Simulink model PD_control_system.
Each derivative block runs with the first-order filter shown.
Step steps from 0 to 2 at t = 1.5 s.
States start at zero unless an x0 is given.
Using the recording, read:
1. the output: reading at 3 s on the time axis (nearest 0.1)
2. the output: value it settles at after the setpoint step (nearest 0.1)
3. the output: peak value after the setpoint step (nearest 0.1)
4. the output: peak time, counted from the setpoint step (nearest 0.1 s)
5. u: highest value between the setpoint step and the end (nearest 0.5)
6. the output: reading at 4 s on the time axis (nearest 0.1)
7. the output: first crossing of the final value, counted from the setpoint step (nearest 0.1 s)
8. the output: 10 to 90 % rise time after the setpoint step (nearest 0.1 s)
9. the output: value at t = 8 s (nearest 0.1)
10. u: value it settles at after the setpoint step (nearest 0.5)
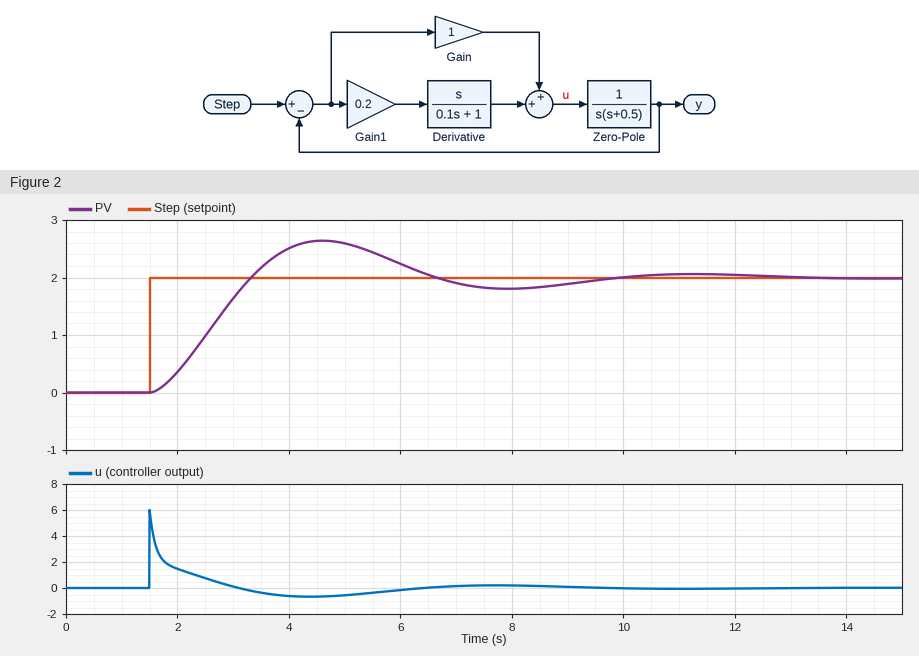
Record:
1.6
2.0
2.6
3.1 s
6.0
2.5
1.8 s
1.3 s
1.8
0.0
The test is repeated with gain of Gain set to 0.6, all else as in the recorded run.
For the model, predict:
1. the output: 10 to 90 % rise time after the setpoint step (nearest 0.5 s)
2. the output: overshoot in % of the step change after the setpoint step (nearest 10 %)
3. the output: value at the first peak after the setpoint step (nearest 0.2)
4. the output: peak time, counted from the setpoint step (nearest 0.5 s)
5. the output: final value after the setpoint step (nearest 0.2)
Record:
2.0 s
20 %
2.4
4.0 s
2.0
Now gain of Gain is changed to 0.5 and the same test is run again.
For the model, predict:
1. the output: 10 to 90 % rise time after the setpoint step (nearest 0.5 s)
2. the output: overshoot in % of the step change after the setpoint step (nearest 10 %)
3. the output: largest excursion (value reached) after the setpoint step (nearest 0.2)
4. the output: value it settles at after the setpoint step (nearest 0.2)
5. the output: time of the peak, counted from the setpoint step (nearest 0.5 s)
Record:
2.0 s
20 %
2.4
2.0
4.5 s
